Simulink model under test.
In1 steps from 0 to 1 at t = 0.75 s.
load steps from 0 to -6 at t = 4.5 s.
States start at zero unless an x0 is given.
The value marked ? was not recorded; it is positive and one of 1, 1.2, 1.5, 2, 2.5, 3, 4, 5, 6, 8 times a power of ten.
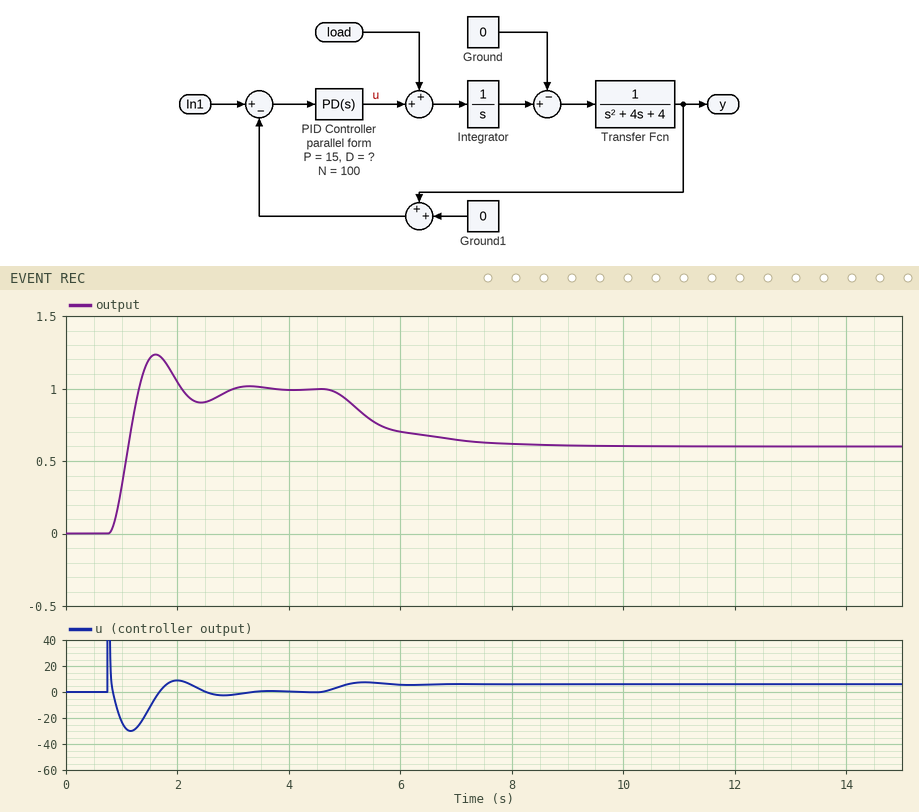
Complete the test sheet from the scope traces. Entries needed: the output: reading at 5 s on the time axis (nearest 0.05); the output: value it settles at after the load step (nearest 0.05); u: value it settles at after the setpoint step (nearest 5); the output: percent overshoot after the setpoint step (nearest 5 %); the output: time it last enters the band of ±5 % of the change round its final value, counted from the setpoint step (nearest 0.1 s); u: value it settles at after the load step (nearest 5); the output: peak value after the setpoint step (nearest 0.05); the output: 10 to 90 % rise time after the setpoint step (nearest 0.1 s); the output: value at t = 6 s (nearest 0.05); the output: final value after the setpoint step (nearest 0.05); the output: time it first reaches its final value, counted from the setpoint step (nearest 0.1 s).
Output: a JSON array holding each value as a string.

["0.95", "0.60", "0", "25 %", "2.0 s", "5", "1.25", "0.4 s", "0.70", "1.00", "0.6 s"]
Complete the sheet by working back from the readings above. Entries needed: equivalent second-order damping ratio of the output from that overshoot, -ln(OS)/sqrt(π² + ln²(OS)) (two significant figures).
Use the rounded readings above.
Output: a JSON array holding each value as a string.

["0.40"]
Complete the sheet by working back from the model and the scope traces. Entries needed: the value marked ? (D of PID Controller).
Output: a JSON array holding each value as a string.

["15"]
